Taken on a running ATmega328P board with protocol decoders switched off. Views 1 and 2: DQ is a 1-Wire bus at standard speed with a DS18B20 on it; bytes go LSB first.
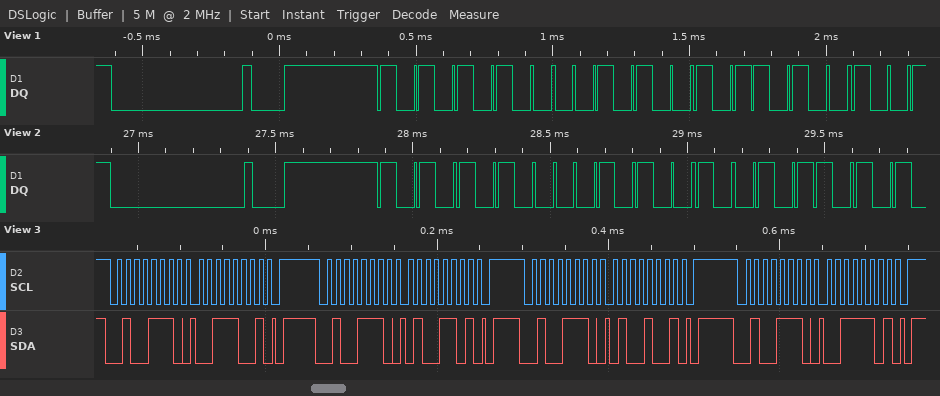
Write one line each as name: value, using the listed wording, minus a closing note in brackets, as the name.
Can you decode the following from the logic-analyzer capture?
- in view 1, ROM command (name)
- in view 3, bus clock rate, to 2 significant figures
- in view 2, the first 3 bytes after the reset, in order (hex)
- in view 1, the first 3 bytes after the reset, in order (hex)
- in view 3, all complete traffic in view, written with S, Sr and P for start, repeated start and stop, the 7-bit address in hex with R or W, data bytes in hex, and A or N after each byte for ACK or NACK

in view 1, ROM command: Match ROM
in view 3, bus clock rate, to 2 significant figures: 100 kHz
in view 2, the first 3 bytes after the reset, in order: 55 28 69
in view 1, the first 3 bytes after the reset, in order: 55 28 2D
in view 3, all complete traffic in view, written with S, Sr and P for start, repeated start and stop, the 7-bit address in hex with R or W, data bytes in hex, and A or N after each byte for ACK or NACK: S 27W A 39 A P S 27W A 4D A P S 27W A 49 A P S 27W A 3D A P
